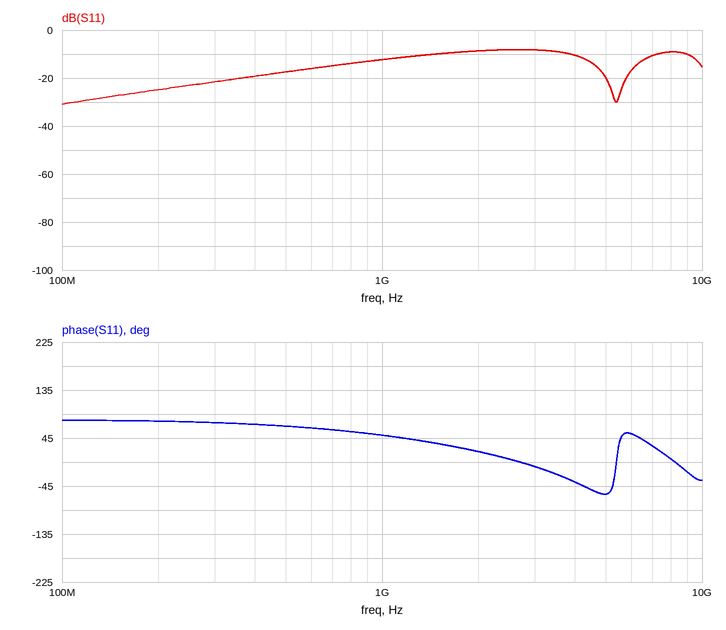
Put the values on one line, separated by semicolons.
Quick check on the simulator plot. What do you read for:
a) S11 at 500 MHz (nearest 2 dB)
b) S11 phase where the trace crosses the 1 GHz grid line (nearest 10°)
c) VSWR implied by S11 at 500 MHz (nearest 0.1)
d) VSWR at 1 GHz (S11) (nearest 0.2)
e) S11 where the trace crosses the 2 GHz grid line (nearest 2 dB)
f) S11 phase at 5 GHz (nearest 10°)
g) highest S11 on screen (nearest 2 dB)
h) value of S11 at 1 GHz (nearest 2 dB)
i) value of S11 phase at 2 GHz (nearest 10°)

-18 dB; 50°; 1.3; 1.6; -8 dB; -60°; -8 dB; -12 dB; 20°
